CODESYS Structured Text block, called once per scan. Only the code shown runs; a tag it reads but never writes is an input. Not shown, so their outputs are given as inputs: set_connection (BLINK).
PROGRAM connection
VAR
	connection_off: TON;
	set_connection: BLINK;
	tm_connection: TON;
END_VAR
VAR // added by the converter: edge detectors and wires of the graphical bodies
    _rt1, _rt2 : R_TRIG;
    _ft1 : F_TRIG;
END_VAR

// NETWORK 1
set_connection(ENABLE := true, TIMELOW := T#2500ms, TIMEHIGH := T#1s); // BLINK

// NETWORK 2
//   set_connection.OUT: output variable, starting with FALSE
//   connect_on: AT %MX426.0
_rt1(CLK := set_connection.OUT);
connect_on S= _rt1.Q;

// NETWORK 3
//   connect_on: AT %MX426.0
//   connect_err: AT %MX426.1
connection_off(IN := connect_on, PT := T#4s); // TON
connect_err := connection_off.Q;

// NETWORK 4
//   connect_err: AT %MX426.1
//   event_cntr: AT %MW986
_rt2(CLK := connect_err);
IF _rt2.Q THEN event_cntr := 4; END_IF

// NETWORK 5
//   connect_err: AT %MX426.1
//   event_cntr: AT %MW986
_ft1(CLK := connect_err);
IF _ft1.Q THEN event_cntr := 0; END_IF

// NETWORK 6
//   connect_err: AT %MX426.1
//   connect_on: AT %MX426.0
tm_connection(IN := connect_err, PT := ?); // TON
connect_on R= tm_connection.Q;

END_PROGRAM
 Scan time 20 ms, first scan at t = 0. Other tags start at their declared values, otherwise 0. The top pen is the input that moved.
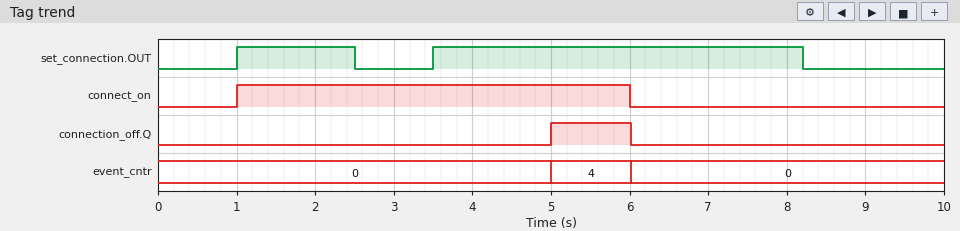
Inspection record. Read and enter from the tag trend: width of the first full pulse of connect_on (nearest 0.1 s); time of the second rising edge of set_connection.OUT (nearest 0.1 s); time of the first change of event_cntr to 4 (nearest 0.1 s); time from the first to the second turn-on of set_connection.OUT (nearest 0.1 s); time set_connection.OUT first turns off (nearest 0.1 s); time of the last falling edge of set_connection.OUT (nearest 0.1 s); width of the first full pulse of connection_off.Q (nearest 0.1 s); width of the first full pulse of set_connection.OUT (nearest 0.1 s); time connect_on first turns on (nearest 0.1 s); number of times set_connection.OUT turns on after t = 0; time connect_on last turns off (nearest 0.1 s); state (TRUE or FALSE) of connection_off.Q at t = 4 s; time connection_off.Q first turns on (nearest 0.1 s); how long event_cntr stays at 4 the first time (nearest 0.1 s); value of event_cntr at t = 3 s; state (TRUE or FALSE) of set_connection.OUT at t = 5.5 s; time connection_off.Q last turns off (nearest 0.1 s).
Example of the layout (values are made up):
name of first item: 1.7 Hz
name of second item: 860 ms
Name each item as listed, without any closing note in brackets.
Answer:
width of the first full pulse of connect_on: 5.0 s
time of the second rising edge of set_connection.OUT: 3.5 s
time of the first change of event_cntr to 4: 5.0 s
time from the first to the second turn-on of set_connection.OUT: 2.5 s
time set_connection.OUT first turns off: 2.5 s
time of the last falling edge of set_connection.OUT: 8.2 s
width of the first full pulse of connection_off.Q: 1.0 s
width of the first full pulse of set_connection.OUT: 1.5 s
time connect_on first turns on: 1.0 s
number of times set_connection.OUT turns on after t = 0: 2
time connect_on last turns off: 6.0 s
state (TRUE or FALSE) of connection_off.Q at t = 4 s: FALSE
time connection_off.Q first turns on: 5.0 s
how long event_cntr stays at 4 the first time: 1.0 s
value of event_cntr at t = 3 s: 0
state (TRUE or FALSE) of set_connection.OUT at t = 5.5 s: TRUE
time connection_off.Q last turns off: 6.0 s
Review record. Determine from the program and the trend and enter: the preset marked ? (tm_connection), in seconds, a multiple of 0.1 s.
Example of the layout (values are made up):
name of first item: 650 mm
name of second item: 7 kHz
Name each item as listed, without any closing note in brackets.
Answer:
the preset marked ? (tm_connection), in seconds, a multiple of 0.1 s: 1.0 s
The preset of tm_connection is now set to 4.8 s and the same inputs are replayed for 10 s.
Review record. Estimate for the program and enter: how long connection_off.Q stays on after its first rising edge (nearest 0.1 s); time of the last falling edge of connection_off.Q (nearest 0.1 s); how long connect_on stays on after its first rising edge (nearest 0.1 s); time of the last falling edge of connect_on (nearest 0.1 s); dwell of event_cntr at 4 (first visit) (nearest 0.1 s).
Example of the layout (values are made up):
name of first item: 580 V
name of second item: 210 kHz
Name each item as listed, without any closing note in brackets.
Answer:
how long connection_off.Q stays on after its first rising edge: 4.8 s
time of the last falling edge of connection_off.Q: 9.8 s
how long connect_on stays on after its first rising edge: 8.8 s
time of the last falling edge of connect_on: 9.8 s
dwell of event_cntr at 4 (first visit): 4.8 s
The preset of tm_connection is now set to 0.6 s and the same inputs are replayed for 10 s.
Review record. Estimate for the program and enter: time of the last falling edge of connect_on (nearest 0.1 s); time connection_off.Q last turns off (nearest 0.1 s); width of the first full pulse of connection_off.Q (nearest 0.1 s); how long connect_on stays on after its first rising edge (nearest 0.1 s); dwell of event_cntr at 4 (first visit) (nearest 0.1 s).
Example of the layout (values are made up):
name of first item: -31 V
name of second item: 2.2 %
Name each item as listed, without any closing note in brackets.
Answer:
time of the last falling edge of connect_on: 5.6 s
time connection_off.Q last turns off: 5.6 s
width of the first full pulse of connection_off.Q: 0.6 s
how long connect_on stays on after its first rising edge: 4.6 s
dwell of event_cntr at 4 (first visit): 0.6 s
